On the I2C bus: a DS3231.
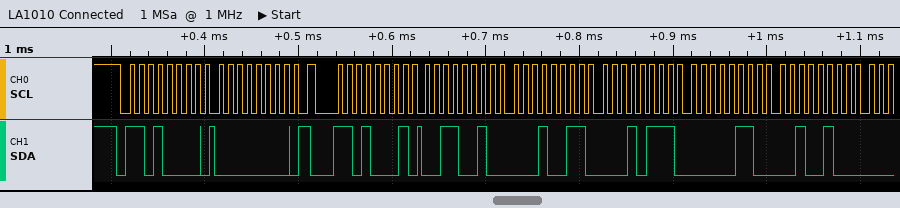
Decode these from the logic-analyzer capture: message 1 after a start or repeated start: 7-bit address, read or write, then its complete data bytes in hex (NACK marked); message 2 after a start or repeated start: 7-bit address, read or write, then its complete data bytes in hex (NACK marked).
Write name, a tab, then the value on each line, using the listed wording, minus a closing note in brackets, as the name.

message 1 after a start or repeated start: 7-bit address, read or write, then its complete data bytes in hex	0x68 write: 00
message 2 after a start or repeated start: 7-bit address, read or write, then its complete data bytes in hex	0x68 read: 32 13 17 06 24
